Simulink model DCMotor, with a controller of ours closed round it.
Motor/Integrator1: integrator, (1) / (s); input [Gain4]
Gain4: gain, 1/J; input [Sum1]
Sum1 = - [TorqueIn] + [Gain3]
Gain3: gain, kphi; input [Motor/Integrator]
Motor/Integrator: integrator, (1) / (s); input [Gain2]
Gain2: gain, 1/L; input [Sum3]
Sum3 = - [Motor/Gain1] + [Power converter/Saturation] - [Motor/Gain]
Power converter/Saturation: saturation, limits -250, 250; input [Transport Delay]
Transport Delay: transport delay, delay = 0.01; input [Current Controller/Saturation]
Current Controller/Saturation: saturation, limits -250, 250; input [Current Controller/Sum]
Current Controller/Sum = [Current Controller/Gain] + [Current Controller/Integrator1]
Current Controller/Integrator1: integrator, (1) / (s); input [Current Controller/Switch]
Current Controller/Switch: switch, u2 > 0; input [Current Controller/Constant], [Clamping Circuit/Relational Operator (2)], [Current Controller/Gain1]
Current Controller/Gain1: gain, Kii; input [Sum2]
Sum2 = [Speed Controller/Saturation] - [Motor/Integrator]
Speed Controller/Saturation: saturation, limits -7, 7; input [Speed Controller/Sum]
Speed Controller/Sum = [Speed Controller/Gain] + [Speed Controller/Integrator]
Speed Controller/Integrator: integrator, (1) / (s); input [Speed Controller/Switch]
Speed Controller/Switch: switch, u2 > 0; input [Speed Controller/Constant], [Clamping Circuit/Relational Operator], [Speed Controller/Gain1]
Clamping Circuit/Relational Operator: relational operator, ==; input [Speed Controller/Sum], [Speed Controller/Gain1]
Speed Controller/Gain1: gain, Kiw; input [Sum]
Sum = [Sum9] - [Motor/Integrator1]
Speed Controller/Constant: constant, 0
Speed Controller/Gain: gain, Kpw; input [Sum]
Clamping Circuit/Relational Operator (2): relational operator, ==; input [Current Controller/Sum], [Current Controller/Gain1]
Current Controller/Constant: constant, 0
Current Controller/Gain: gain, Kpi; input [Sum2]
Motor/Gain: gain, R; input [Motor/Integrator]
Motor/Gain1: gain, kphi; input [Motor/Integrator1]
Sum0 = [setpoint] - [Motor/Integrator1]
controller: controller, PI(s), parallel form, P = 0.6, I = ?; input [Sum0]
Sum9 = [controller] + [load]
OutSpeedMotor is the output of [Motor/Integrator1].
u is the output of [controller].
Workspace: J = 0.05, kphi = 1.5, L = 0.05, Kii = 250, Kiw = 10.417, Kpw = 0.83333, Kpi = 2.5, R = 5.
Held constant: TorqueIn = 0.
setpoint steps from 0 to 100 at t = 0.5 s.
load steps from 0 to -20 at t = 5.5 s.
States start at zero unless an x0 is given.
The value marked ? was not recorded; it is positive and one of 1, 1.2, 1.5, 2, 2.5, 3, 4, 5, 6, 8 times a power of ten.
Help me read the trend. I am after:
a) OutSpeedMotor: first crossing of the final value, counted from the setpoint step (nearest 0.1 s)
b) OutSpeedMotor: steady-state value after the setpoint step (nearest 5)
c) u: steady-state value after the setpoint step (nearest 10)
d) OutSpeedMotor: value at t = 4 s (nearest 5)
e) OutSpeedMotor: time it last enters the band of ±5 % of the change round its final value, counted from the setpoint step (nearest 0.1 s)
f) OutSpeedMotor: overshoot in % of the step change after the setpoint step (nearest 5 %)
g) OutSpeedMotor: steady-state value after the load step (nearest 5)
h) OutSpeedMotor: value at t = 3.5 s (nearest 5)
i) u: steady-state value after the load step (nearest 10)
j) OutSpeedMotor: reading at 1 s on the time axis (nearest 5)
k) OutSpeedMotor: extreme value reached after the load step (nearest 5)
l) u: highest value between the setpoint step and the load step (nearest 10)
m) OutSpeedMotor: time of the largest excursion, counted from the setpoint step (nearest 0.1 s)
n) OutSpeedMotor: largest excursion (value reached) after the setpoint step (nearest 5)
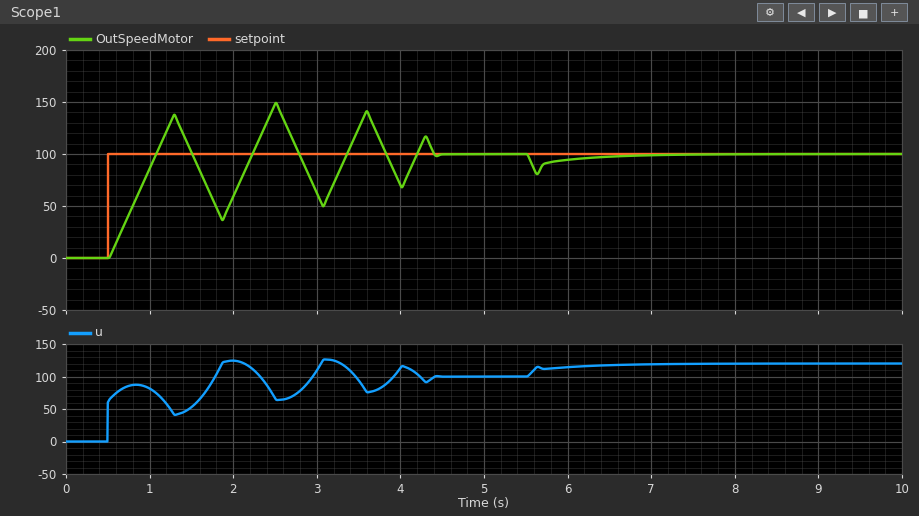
0.6 s
100
100
70
3.9 s
50 %
100
125
120
85
80
130
2.0 s
150
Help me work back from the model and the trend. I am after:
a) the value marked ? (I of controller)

2.5
